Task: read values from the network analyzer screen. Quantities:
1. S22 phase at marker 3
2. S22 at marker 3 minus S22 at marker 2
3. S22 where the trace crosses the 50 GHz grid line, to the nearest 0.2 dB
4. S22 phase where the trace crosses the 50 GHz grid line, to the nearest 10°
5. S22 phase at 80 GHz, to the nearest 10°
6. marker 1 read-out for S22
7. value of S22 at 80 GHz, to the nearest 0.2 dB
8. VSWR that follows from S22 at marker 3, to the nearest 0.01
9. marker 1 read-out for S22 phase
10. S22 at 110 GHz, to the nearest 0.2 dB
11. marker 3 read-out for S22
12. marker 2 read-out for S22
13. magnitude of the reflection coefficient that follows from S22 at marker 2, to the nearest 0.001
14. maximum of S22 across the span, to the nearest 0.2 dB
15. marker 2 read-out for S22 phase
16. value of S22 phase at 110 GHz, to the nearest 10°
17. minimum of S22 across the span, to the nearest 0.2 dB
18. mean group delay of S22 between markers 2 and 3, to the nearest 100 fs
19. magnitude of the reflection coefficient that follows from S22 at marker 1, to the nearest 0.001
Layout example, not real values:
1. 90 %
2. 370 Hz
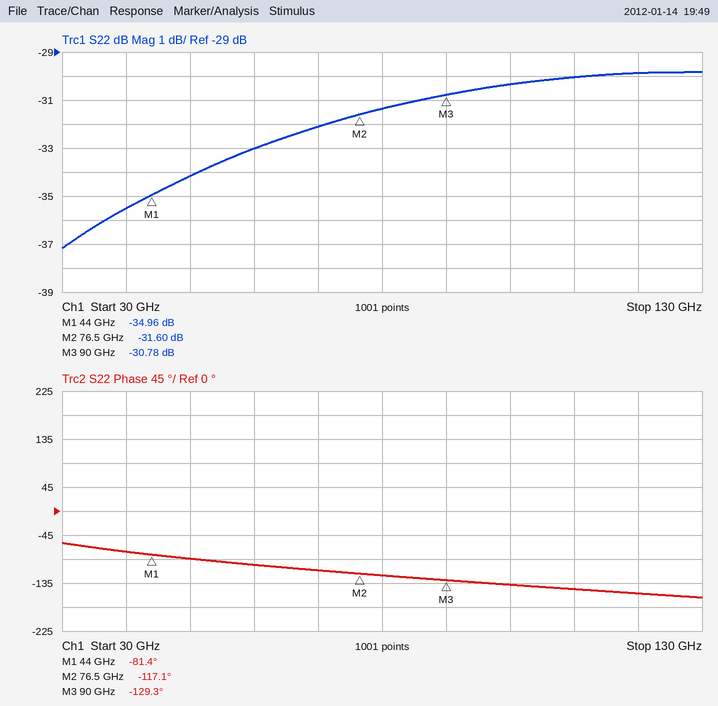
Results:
1. -129.3°
2. 0.82 dB
3. -34.2 dB
4. -90°
5. -120°
6. -34.96 dB
7. -31.4 dB
8. 1.06
9. -81.4°
10. -30.0 dB
11. -30.78 dB
12. -31.60 dB
13. 0.026
14. -29.8 dB
15. -117.1°
16. -150°
17. -37.2 dB
18. 2.5 ps
19. 0.018
